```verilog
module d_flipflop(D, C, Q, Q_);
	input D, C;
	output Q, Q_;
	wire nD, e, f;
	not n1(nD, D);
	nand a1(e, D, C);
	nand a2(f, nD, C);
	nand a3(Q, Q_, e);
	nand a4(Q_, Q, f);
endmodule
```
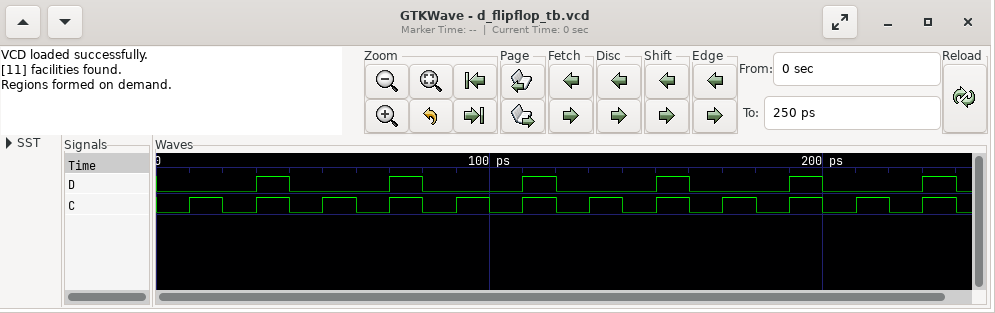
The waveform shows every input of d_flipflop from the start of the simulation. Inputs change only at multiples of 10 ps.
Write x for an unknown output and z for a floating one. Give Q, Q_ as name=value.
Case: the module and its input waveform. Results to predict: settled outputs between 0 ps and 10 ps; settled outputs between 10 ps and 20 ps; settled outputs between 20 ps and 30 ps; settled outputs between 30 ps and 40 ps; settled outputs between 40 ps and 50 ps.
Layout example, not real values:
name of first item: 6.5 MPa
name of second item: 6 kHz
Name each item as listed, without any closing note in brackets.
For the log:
settled outputs between 0 ps and 10 ps: Q=x, Q_=x
settled outputs between 10 ps and 20 ps: Q=0, Q_=1
settled outputs between 20 ps and 30 ps: Q=0, Q_=1
settled outputs between 30 ps and 40 ps: Q=1, Q_=0
settled outputs between 40 ps and 50 ps: Q=1, Q_=0
